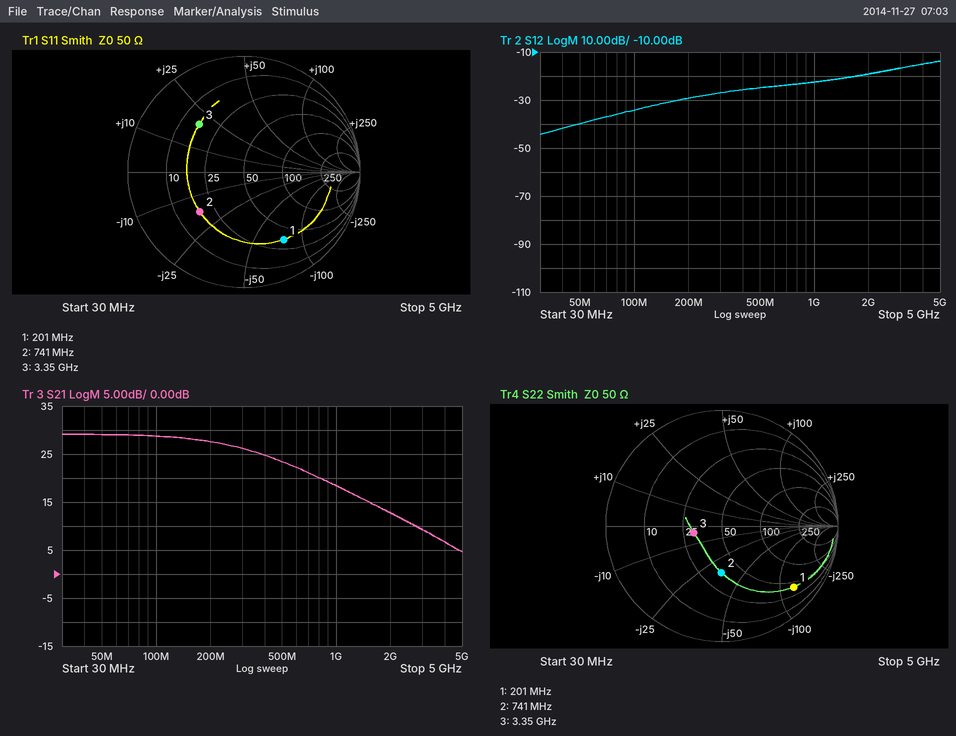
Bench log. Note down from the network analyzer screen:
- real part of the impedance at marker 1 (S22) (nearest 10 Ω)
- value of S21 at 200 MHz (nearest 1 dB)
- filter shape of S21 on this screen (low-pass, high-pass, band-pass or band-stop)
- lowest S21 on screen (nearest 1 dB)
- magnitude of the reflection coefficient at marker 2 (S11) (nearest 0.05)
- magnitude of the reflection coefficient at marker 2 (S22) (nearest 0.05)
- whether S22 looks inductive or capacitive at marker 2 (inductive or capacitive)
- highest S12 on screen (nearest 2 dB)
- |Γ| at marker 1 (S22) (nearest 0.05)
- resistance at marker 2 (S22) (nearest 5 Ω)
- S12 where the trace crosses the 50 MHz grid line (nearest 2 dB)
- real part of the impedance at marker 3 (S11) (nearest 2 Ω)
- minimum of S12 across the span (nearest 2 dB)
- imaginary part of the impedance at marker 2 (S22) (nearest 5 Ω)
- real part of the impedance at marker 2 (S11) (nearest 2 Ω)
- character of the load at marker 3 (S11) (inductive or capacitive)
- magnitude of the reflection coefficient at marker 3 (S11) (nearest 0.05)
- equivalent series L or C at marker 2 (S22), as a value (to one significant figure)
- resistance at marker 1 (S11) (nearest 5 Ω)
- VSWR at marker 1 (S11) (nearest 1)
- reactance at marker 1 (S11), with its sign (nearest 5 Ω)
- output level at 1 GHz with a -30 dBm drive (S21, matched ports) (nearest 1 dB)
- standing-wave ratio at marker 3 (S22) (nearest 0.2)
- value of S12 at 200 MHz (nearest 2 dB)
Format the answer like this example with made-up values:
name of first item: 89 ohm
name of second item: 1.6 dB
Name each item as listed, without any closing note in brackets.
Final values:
real part of the impedance at marker 1 (S22): 40 Ω
value of S21 at 200 MHz: 28 dB
filter shape of S21 on this screen: low-pass
lowest S21 on screen: 5 dB
magnitude of the reflection coefficient at marker 2 (S11): 0.50
magnitude of the reflection coefficient at marker 2 (S22): 0.40
whether S22 looks inductive or capacitive at marker 2: capacitive
highest S12 on screen: -14 dB
|Γ| at marker 1 (S22): 0.80
resistance at marker 2 (S22): 35 Ω
S12 where the trace crosses the 50 MHz grid line: -40 dB
real part of the impedance at marker 3 (S11): 16 Ω
minimum of S12 across the span: -44 dB
imaginary part of the impedance at marker 2 (S22): -35 Ω
real part of the impedance at marker 2 (S11): 18 Ω
character of the load at marker 3 (S11): inductive
magnitude of the reflection coefficient at marker 3 (S11): 0.55
equivalent series L or C at marker 2 (S22), as a value: 6 pF
resistance at marker 1 (S11): 35 Ω
VSWR at marker 1 (S11): 5
reactance at marker 1 (S11), with its sign: -75 Ω
output level at 1 GHz with a -30 dBm drive (S21, matched ports): -12 dBm
standing-wave ratio at marker 3 (S22): 1.6
value of S12 at 200 MHz: -30 dB
